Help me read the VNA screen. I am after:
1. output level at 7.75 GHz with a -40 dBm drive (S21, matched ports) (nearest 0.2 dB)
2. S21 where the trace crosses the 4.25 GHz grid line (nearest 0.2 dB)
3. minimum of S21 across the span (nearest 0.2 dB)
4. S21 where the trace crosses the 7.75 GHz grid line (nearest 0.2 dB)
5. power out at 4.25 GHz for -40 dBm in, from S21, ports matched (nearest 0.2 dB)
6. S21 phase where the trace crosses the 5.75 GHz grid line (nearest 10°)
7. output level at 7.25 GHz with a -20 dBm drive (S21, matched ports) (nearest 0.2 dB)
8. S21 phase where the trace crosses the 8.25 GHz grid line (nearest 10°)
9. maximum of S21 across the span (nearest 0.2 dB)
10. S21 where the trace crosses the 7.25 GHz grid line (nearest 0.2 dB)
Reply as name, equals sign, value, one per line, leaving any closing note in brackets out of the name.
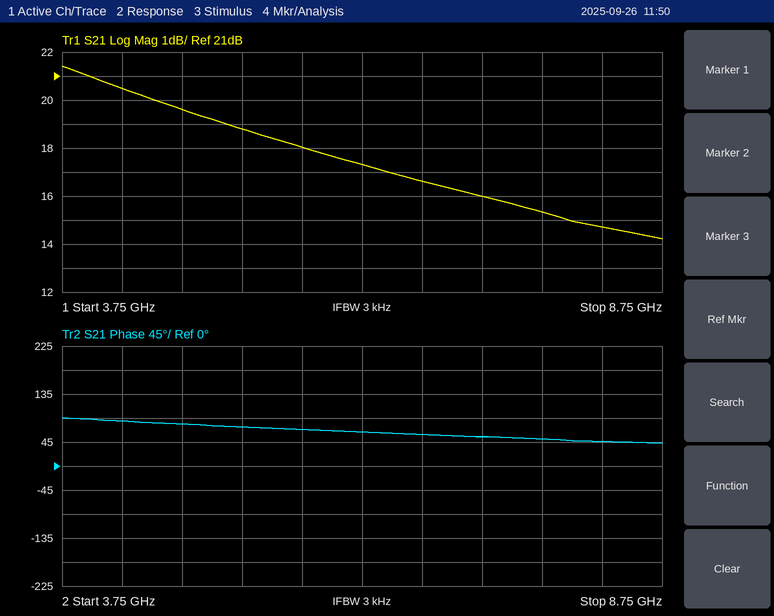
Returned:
output level at 7.75 GHz with a -40 dBm drive (S21, matched ports) = -24.6 dBm
S21 where the trace crosses the 4.25 GHz grid line = 20.4 dB
minimum of S21 across the span = 14.2 dB
S21 where the trace crosses the 7.75 GHz grid line = 15.4 dB
power out at 4.25 GHz for -40 dBm in, from S21, ports matched = -19.6 dBm
S21 phase where the trace crosses the 5.75 GHz grid line = 70°
output level at 7.25 GHz with a -20 dBm drive (S21, matched ports) = -4.0 dBm
S21 phase where the trace crosses the 8.25 GHz grid line = 50°
maximum of S21 across the span = 21.4 dB
S21 where the trace crosses the 7.25 GHz grid line = 16.0 dB
